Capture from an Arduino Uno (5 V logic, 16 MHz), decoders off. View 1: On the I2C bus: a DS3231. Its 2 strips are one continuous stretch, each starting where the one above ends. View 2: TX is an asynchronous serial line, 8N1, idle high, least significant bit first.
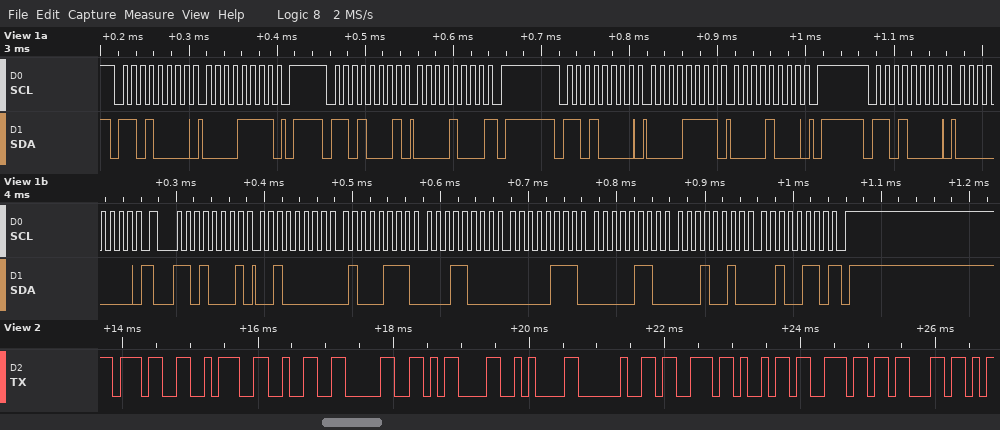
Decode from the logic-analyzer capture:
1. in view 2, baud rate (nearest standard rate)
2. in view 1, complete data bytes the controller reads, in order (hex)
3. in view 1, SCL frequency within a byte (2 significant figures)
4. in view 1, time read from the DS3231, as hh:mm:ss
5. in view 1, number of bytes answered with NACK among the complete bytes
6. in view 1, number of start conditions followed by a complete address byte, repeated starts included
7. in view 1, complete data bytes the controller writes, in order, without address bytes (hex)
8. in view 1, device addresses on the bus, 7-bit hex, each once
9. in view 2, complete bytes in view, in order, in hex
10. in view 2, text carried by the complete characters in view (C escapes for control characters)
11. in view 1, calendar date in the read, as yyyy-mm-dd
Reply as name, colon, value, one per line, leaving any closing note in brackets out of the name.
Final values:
in view 2, baud rate: 9600 baud
in view 1, complete data bytes the controller reads, in order: 08 20 47 18 07 06 12 26
in view 1, SCL frequency within a byte: 100 kHz
in view 1, time read from the DS3231, as hh:mm:ss: 18:47:20
in view 1, number of bytes answered with NACK among the complete bytes: 2
in view 1, number of start conditions followed by a complete address byte, repeated starts included: 5
in view 1, complete data bytes the controller writes, in order, without address bytes: 0F 0F 08 00
in view 1, device addresses on the bus, 7-bit hex, each once: 0x68
in view 2, complete bytes in view, in order, in hex: 37 3A 32 30 0D 0A 20 73 69 6E 63
in view 2, text carried by the complete characters in view: "7:20\r\n sinc"
in view 1, calendar date in the read, as yyyy-mm-dd: 2026-12-06
